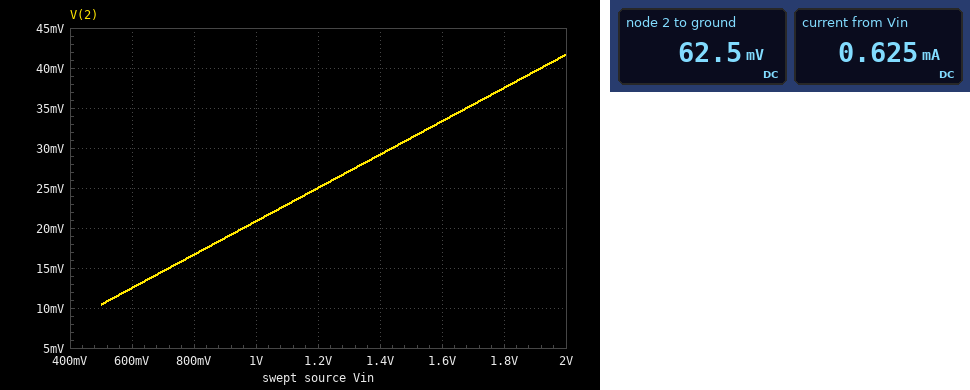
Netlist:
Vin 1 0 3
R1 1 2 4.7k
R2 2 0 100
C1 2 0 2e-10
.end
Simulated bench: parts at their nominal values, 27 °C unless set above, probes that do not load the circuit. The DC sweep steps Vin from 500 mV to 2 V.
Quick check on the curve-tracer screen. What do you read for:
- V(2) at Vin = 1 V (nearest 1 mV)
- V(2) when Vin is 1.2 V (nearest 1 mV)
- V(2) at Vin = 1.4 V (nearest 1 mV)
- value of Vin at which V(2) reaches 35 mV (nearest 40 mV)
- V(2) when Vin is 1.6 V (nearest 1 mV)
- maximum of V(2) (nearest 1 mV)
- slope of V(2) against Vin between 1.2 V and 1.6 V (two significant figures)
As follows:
21 mV
25 mV
29 mV
1.68 V
33 mV
42 mV
0.021 V/V
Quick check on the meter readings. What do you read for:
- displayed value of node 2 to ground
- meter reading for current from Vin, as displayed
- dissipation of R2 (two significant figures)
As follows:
62.5 mV
0.625 mA
39 µW
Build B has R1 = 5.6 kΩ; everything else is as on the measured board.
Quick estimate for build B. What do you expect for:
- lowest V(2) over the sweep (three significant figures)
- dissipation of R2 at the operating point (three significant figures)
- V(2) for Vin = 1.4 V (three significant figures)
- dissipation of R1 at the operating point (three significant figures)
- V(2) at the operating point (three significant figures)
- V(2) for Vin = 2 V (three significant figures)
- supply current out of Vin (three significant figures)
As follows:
8.77 mV
27.7 µW
24.6 mV
1.55 mW
52.6 mV
35.1 mV
526 µA
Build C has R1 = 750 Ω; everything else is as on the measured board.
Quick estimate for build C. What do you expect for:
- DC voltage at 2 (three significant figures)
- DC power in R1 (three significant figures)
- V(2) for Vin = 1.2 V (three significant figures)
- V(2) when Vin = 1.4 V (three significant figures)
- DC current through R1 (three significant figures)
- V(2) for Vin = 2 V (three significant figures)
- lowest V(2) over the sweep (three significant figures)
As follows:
353 mV
9.34 mW
141 mV
165 mV
3.53 mA
235 mV
58.8 mV
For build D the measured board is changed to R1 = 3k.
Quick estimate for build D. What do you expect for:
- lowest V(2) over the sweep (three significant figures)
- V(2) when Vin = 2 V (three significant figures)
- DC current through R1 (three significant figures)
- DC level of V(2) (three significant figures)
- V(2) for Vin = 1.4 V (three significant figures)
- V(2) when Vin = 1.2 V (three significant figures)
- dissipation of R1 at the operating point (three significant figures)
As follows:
16.1 mV
64.5 mV
968 µA
96.8 mV
45.2 mV
38.7 mV
2.81 mW
